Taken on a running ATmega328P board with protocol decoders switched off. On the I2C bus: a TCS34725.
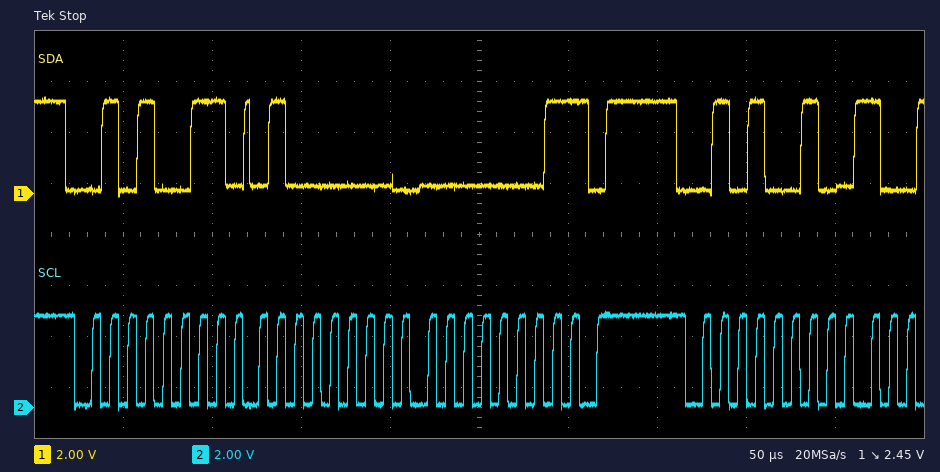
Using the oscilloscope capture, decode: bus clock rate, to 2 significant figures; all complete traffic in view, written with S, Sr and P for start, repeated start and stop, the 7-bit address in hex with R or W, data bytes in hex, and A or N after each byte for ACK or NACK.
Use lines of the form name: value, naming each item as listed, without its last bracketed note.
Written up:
bus clock rate, to 2 significant figures: 100 kHz
all complete traffic in view, written with S, Sr and P for start, repeated start and stop, the 7-bit address in hex with R or W, data bytes in hex, and A or N after each byte for ACK or NACK: S 29R A 40 A 01 N P S 29W A
